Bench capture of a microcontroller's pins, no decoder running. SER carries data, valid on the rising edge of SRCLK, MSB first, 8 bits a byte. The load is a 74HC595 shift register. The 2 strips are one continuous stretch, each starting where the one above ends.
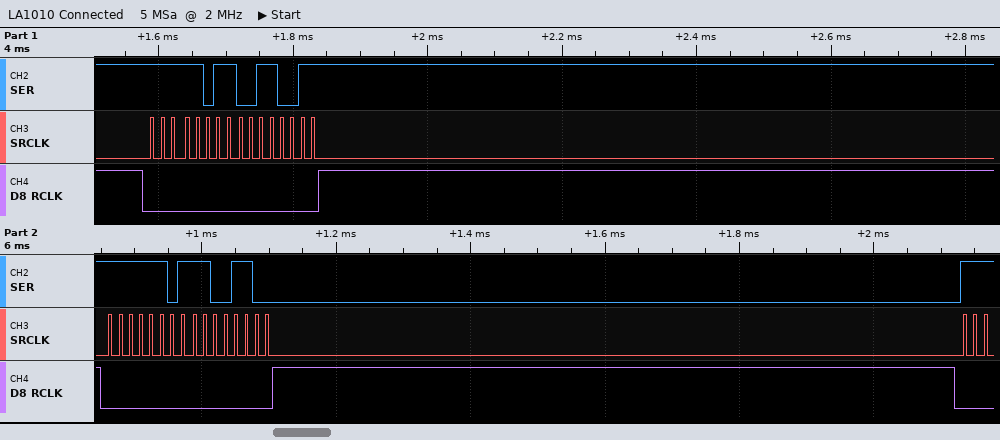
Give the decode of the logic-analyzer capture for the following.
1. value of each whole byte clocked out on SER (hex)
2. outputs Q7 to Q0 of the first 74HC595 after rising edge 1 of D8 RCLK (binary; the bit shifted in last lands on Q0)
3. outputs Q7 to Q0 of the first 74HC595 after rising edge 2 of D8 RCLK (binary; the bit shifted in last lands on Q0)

0xFB 0x33 0xFD 0xCC
00110011
11001100
